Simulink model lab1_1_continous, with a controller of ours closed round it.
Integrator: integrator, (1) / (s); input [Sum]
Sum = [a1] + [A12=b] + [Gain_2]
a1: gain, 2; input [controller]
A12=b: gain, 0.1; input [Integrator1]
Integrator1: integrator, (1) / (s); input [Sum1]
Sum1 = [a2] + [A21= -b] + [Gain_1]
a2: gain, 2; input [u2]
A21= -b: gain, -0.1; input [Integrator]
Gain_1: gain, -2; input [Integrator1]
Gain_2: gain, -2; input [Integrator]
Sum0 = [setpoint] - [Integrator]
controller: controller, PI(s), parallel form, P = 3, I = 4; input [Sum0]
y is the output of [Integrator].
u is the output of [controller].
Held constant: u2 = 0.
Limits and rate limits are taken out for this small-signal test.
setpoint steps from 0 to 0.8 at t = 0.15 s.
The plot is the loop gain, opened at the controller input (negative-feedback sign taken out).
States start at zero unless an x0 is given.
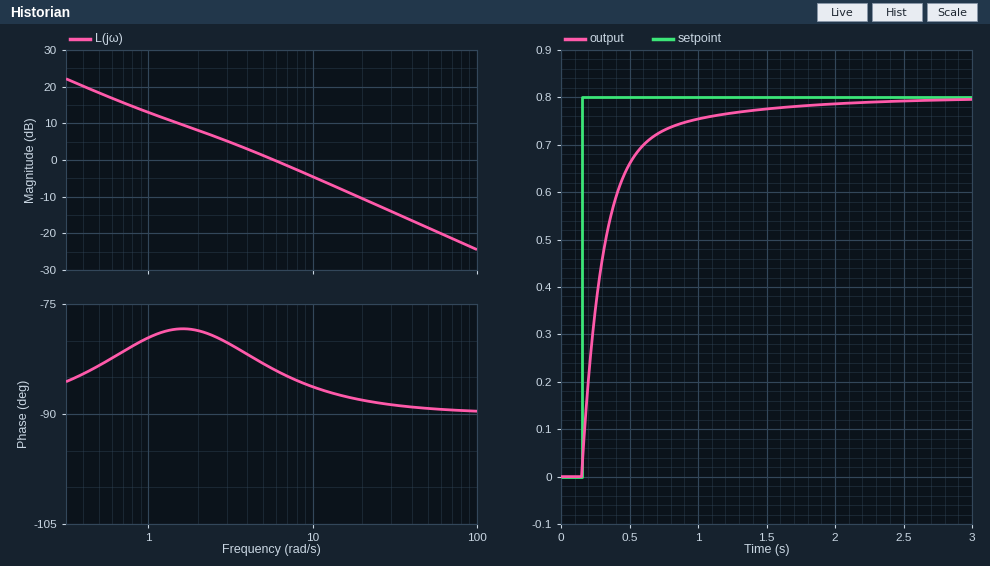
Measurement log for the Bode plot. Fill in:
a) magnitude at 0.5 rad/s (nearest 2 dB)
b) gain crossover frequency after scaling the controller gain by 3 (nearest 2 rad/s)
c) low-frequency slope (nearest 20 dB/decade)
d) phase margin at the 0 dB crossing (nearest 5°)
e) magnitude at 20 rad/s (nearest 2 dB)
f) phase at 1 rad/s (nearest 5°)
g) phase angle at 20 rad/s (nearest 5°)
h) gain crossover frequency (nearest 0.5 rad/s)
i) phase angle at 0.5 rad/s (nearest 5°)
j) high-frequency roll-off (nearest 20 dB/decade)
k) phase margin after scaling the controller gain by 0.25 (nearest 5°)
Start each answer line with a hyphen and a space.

- 18 dB
- 18 rad/s
- -20 dB/decade
- 95°
- -10 dB
- -80°
- -90°
- 6.0 rad/s
- -85°
- -20 dB/decade
- 100°
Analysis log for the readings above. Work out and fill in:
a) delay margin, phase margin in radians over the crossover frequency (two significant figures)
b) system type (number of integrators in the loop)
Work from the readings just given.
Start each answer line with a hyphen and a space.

- 0.28 s
- 1
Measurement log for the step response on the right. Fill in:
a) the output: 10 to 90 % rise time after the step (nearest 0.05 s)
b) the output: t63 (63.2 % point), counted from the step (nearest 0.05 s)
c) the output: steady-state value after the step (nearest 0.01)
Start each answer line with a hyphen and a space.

- 0.50 s
- 0.20 s
- 0.80
